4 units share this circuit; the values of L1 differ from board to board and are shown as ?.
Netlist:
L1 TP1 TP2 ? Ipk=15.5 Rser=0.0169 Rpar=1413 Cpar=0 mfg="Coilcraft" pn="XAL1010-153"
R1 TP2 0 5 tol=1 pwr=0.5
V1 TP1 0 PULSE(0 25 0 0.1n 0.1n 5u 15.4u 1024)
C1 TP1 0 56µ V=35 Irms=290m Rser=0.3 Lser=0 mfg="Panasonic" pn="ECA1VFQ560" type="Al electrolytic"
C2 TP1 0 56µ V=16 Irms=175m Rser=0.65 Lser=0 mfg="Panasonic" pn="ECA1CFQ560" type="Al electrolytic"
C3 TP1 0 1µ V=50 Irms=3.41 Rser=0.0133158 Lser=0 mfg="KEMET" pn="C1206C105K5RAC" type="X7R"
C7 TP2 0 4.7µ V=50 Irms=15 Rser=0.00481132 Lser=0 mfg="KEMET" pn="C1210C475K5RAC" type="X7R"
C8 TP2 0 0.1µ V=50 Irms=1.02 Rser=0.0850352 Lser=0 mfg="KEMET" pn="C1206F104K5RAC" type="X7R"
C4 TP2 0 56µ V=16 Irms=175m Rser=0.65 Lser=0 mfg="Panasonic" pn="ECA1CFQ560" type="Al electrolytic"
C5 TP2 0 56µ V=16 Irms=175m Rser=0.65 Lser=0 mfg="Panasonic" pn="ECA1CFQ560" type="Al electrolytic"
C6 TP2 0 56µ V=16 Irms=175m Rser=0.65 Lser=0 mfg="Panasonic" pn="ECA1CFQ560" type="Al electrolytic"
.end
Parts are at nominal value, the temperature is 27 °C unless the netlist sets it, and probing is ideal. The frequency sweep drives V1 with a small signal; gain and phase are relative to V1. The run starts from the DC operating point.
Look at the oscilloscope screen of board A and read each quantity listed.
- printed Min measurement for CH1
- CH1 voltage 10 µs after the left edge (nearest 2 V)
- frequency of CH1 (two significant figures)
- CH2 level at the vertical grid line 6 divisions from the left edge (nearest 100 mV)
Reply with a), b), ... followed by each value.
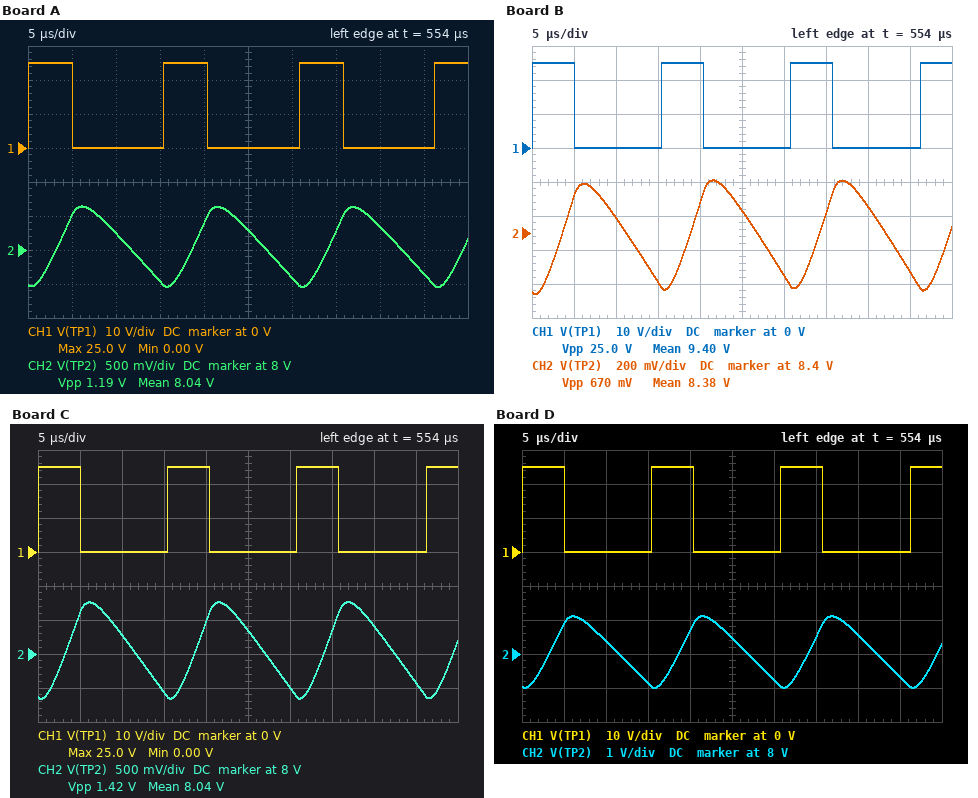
a) 0.00 V
b) 0 V
c) 65 kHz
d) 7.6 V
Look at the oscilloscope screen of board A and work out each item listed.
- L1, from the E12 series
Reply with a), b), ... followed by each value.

a) 12 µH
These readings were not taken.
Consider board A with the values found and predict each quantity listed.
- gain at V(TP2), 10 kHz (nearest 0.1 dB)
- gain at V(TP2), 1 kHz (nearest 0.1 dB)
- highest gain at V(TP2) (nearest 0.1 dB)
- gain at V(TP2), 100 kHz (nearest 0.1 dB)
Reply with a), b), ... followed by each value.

a) -9.9 dB
b) 0.6 dB
c) 3.5 dB
d) -32.7 dB
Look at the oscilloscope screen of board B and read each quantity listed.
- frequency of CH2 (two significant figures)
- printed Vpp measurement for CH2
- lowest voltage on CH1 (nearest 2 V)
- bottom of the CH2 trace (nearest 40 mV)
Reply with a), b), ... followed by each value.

a) 65 kHz
b) 670 mV
c) 0 V
d) 8.04 V
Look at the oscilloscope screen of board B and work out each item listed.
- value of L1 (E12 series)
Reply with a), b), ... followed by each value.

a) 22 µH
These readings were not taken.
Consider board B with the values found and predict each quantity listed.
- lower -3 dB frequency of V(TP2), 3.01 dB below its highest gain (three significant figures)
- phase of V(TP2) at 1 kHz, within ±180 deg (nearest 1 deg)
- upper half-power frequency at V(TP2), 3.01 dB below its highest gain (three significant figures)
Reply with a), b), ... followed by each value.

a) 1.22 kHz
b) -5 deg
c) 3.14 kHz
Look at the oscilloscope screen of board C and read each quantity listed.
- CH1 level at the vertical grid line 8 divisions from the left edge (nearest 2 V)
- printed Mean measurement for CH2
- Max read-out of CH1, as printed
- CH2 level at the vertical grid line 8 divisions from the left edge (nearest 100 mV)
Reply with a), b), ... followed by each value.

a) 0 V
b) 8.04 V
c) 25.0 V
d) 8.4 V
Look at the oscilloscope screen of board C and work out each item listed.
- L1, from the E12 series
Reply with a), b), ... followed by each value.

a) 10 µH
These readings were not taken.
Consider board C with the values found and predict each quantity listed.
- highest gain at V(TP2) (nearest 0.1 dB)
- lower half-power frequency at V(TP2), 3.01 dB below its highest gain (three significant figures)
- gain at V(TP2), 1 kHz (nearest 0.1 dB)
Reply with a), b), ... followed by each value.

a) 3.1 dB
b) 530 Hz
c) 0.5 dB
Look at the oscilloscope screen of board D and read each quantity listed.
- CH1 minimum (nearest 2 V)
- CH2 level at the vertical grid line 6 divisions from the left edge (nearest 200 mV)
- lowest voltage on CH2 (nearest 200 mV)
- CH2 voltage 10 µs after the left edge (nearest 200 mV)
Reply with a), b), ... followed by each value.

a) 0 V
b) 7.2 V
c) 7.0 V
d) 8.4 V
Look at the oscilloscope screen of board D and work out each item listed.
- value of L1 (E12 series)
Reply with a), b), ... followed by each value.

a) 6.8 µH
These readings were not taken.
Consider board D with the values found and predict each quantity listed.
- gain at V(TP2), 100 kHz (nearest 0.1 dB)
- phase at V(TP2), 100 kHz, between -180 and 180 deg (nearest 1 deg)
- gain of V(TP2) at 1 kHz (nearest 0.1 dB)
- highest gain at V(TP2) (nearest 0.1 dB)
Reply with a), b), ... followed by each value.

a) -27.7 dB
b) -121 deg
c) 0.3 dB
d) 2.4 dB
